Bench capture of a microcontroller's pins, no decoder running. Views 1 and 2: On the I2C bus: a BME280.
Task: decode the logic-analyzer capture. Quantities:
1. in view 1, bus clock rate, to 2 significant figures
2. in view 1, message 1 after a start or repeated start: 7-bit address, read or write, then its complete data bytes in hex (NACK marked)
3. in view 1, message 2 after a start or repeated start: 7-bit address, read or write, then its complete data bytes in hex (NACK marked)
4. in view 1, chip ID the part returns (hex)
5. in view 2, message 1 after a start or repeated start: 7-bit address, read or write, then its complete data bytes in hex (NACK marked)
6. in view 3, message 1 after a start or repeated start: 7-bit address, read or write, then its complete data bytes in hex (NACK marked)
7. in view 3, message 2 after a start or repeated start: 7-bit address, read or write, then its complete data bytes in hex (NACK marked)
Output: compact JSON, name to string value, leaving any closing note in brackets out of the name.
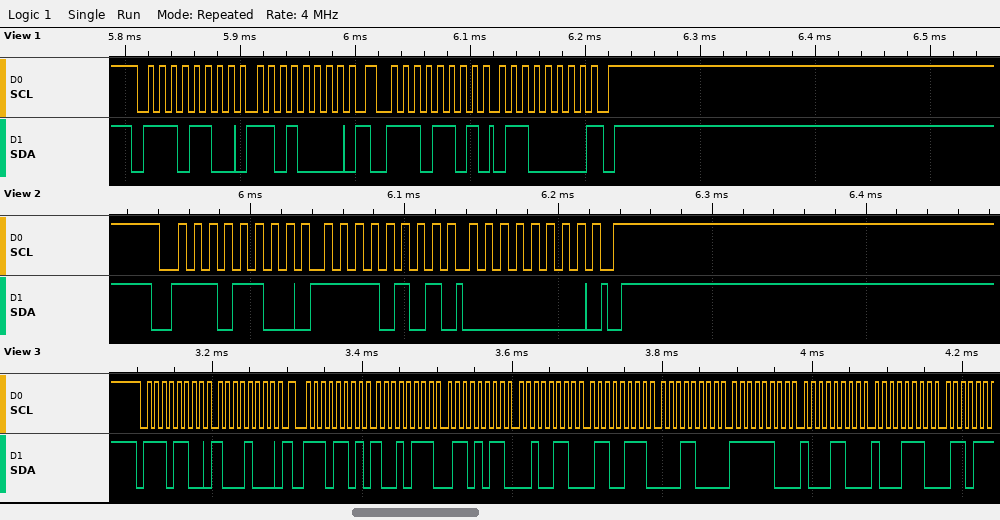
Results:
{"in view 1, bus clock rate, to 2 significant figures": "100 kHz", "in view 1, message 1 after a start or repeated start: 7-bit address, read or write, then its complete data bytes in hex": "0x76 write: D0", "in view 1, message 2 after a start or repeated start: 7-bit address, read or write, then its complete data bytes in hex": "0x76 read: 60 NACK", "in view 1, chip ID the part returns": "0x60", "in view 2, message 1 after a start or repeated start: 7-bit address, read or write, then its complete data bytes in hex": "0x76 write: F5 00", "in view 3, message 1 after a start or repeated start: 7-bit address, read or write, then its complete data bytes in hex": "0x76 write: 88", "in view 3, message 2 after a start or repeated start: 7-bit address, read or write, then its complete data bytes in hex": "0x76 read: 97 6B 26 67 18 FC 8C 8E"}
